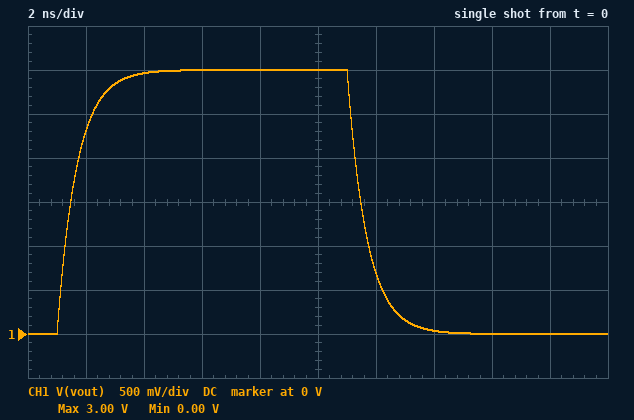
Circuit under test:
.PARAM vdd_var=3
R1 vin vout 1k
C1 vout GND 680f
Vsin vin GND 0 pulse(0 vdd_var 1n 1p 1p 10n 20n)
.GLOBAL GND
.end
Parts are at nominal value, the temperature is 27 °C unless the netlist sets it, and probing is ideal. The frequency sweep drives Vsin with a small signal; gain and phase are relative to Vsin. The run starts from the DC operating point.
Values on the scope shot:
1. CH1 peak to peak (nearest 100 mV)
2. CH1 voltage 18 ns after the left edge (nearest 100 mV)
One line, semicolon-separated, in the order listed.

3.0 V; 0 V
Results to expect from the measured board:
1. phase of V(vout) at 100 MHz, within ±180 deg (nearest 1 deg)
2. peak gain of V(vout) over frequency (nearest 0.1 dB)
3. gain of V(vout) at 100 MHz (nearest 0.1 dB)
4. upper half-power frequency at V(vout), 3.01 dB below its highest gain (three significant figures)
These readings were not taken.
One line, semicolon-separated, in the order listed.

-23 deg; 0 dB; -0.7 dB; 234 MHz
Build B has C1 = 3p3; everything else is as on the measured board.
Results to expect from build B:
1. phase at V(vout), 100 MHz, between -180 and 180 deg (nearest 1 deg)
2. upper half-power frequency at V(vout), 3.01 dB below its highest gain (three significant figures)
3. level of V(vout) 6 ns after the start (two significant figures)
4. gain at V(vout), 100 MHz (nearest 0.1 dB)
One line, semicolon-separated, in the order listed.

-64 deg; 48.2 MHz; 2.3 V; -7.2 dB
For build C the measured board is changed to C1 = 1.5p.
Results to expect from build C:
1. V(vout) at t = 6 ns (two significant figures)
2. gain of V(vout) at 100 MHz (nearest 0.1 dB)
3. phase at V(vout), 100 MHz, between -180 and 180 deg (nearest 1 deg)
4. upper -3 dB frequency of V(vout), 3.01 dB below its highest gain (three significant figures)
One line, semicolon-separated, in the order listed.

2.9 V; -2.8 dB; -43 deg; 106 MHz
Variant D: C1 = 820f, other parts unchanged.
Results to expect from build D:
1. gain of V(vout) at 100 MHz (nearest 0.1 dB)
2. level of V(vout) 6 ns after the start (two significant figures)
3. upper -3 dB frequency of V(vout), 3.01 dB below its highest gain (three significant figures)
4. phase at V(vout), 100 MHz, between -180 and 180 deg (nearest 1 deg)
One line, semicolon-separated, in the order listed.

-1.0 dB; 3.0 V; 194 MHz; -27 deg
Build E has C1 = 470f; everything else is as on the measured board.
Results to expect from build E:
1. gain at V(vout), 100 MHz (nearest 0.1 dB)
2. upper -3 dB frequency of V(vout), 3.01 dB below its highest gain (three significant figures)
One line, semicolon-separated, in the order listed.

-0.4 dB; 339 MHz
